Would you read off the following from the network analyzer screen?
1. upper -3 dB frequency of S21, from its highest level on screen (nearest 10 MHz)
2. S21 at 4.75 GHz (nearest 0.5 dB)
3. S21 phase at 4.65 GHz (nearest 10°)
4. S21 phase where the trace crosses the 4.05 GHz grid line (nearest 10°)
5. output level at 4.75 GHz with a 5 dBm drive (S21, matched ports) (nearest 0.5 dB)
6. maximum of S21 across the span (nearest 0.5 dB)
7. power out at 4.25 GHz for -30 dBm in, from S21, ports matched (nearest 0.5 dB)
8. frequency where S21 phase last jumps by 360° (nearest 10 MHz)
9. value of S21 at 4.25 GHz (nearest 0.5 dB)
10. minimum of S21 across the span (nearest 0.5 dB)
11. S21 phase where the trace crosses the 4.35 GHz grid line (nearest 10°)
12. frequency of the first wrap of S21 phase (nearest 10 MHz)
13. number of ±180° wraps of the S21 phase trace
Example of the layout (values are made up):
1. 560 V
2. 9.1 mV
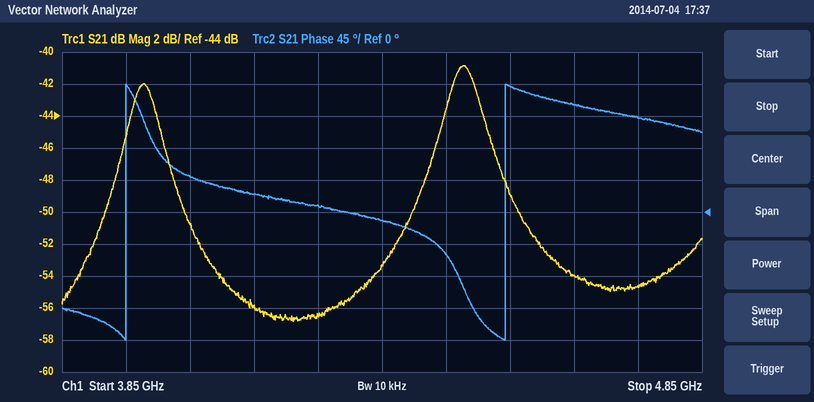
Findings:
1. 4.51 GHz
2. -54.5 dB
3. 150°
4. 50°
5. -49.5 dBm
6. -41.0 dB
7. -86.5 dBm
8. 4.54 GHz
9. -56.5 dB
10. -57.0 dB
11. -10°
12. 3.95 GHz
13. 2
